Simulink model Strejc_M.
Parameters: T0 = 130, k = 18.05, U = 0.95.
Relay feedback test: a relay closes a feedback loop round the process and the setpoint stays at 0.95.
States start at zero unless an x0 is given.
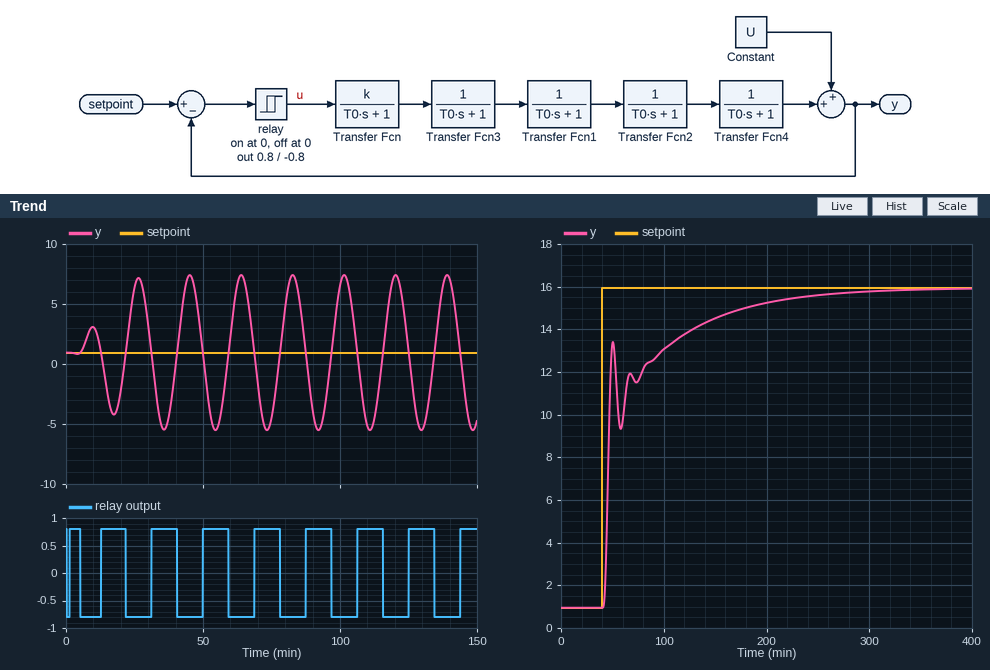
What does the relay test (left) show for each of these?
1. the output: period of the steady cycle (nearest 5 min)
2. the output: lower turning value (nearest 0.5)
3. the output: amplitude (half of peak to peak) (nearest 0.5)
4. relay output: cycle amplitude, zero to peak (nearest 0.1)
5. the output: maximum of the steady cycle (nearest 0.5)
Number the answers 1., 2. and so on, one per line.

1. 20 min
2. -5.5
3. 6.5
4. 0.8
5. 7.5
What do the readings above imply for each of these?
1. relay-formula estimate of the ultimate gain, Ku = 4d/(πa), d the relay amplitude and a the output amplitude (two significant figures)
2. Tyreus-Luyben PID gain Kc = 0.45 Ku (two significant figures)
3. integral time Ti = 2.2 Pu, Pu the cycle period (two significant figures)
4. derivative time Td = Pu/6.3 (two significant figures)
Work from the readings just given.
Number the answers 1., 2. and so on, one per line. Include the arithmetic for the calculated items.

1. 4 × 0.8 / (π × 6.5) = 0.16
2. 0.45 × 0.16 = 0.072
3. 2.2 × 20 = 44 min
4. 20 / 6.3 = 3.2 min
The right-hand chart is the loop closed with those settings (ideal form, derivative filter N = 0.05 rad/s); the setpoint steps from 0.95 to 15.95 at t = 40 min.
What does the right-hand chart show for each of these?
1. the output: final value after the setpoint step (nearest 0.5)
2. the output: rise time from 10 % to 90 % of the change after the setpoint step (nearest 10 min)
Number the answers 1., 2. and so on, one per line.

1. 16.0
2. 100 min
